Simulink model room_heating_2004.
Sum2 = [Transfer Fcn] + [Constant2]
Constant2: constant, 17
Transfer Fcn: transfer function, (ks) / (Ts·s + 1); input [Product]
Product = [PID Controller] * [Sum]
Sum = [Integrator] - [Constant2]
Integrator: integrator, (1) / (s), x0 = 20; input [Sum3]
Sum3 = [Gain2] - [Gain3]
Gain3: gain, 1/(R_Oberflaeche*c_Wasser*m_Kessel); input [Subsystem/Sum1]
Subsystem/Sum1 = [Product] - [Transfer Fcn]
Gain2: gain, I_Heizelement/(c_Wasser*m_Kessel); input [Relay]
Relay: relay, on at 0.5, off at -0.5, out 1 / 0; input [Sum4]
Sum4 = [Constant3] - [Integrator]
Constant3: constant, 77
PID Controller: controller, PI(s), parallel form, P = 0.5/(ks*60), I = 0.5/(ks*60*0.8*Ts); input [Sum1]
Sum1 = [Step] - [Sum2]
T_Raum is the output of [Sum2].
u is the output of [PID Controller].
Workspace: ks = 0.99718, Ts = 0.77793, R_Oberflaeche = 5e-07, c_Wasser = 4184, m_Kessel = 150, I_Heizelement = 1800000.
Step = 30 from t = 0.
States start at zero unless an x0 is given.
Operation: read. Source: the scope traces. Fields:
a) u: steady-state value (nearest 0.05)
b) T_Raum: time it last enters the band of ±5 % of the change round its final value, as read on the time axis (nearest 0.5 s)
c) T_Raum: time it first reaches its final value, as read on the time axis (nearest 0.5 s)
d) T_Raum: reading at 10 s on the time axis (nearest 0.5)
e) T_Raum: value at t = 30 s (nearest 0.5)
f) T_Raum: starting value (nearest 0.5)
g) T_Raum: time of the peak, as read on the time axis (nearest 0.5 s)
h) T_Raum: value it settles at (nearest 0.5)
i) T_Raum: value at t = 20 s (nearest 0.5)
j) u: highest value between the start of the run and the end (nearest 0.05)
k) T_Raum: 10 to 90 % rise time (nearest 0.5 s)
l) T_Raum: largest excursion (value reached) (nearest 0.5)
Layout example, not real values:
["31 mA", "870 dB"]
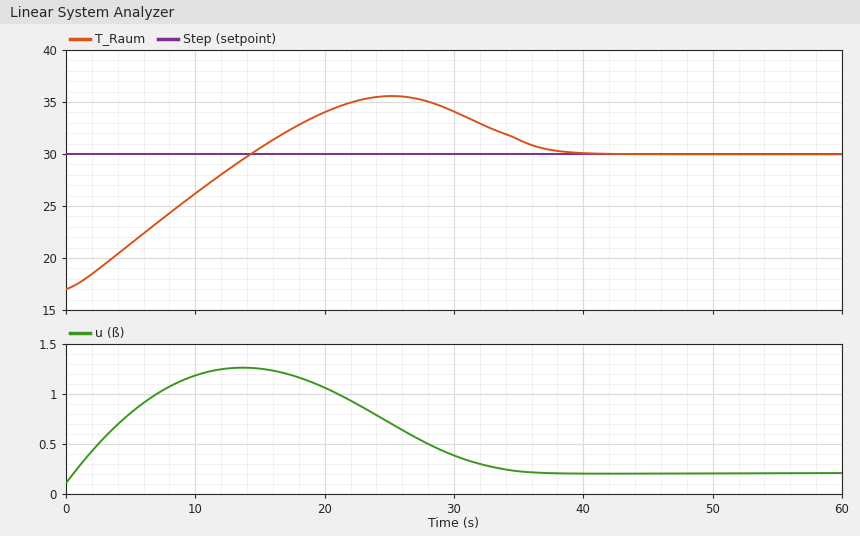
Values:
["0.20", "36.5 s", "14.5 s", "26.0", "34.0", "17.0", "25.0 s", "30.0", "34.0", "1.25", "11.0 s", "35.5"]
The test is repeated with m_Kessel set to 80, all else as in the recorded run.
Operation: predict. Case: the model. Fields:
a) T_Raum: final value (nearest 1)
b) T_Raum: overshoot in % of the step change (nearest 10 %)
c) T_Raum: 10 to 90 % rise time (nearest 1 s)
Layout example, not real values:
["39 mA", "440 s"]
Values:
["30", "50 %", "10 s"]
